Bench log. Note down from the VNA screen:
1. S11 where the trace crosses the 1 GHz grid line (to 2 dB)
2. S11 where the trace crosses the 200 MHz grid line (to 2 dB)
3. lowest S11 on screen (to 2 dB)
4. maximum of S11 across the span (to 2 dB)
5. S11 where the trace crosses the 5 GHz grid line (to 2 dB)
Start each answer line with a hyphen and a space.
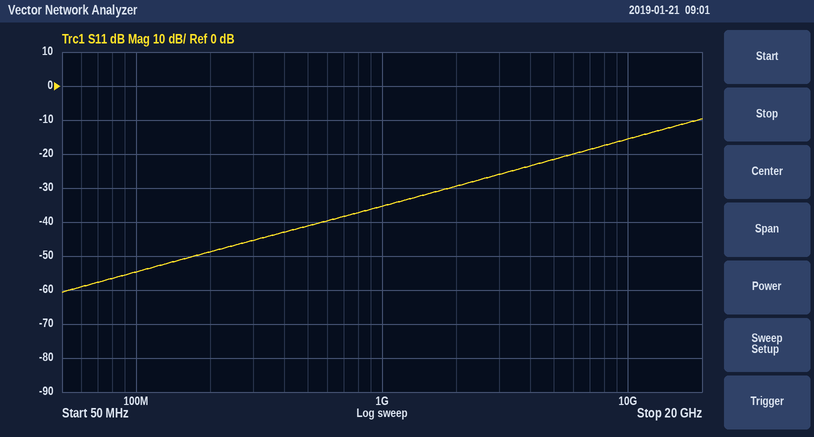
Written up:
- -36 dB
- -48 dB
- -60 dB
- -10 dB
- -22 dB
